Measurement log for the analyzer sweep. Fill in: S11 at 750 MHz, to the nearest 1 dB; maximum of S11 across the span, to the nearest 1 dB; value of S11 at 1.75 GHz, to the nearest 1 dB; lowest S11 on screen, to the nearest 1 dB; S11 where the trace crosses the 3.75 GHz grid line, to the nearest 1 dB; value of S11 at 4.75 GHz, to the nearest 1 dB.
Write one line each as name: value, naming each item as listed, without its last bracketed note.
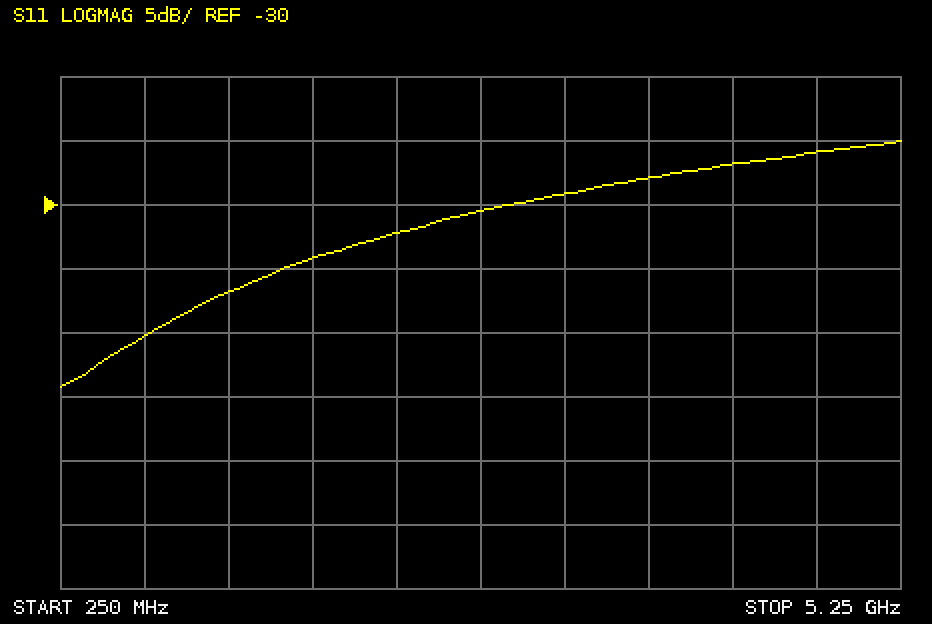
S11 at 750 MHz, to the nearest 1 dB: -40 dB
maximum of S11 across the span, to the nearest 1 dB: -25 dB
value of S11 at 1.75 GHz, to the nearest 1 dB: -34 dB
lowest S11 on screen, to the nearest 1 dB: -44 dB
S11 where the trace crosses the 3.75 GHz grid line, to the nearest 1 dB: -28 dB
value of S11 at 4.75 GHz, to the nearest 1 dB: -26 dB
